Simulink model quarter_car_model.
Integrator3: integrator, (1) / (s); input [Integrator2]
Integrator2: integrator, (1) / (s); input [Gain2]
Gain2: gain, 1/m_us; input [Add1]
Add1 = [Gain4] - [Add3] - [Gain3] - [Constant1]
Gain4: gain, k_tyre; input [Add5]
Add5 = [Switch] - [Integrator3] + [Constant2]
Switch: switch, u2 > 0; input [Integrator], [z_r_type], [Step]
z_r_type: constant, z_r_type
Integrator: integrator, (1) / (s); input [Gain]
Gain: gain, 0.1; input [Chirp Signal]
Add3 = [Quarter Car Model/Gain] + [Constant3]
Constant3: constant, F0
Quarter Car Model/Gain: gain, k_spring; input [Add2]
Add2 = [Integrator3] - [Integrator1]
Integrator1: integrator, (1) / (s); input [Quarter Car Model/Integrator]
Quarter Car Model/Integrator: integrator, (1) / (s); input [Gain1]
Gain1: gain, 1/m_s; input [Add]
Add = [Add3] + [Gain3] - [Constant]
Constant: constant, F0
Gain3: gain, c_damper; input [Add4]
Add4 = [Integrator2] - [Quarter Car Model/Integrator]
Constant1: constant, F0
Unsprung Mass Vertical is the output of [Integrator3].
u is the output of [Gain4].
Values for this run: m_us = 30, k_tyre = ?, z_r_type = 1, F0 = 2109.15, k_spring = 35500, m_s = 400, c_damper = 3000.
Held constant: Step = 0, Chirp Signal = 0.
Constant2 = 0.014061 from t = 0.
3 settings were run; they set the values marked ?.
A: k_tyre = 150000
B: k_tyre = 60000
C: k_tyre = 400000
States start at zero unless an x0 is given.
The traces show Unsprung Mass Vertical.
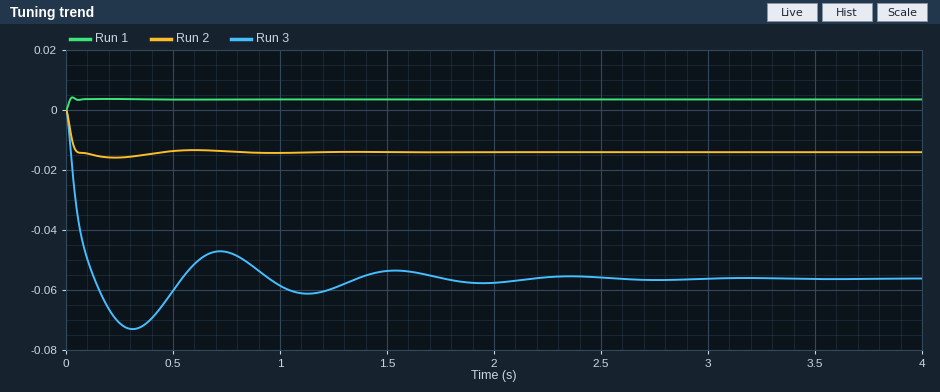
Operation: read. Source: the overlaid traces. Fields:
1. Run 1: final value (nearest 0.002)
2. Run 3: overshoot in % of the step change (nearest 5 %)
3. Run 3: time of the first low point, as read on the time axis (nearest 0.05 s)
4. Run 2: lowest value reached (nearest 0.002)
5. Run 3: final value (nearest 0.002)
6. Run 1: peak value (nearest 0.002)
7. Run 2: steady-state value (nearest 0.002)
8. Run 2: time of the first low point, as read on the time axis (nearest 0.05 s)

0.004
30 %
0.30 s
-0.016
-0.056
0.004
-0.014
0.25 s
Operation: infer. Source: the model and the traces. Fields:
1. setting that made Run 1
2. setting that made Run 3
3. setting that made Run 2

C
B
A
